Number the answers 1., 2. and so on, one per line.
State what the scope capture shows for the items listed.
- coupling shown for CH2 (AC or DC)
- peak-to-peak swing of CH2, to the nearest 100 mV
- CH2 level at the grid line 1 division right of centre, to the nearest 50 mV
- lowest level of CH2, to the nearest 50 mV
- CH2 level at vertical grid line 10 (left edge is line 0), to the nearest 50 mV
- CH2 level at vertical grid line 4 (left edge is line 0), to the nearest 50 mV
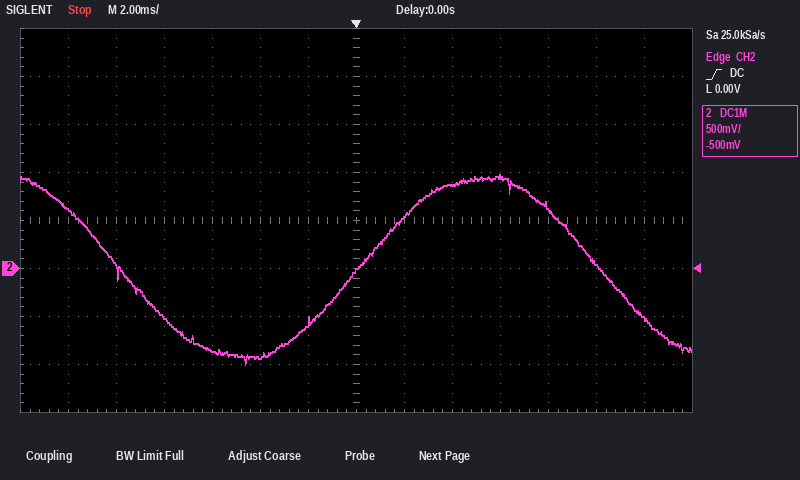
1. DC
2. 2.00 V
3. 550 mV
4. -1.00 V
5. 950 mV
6. -850 mV
